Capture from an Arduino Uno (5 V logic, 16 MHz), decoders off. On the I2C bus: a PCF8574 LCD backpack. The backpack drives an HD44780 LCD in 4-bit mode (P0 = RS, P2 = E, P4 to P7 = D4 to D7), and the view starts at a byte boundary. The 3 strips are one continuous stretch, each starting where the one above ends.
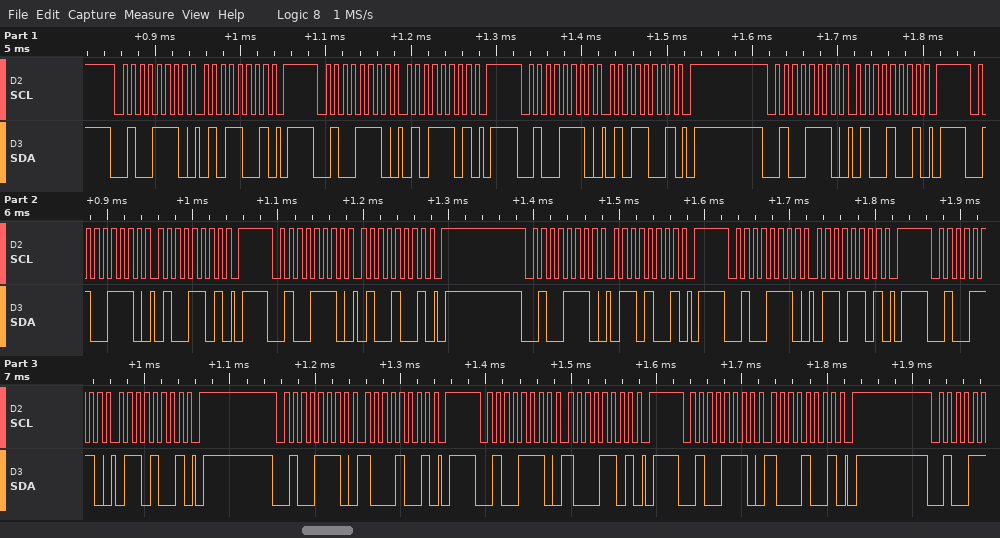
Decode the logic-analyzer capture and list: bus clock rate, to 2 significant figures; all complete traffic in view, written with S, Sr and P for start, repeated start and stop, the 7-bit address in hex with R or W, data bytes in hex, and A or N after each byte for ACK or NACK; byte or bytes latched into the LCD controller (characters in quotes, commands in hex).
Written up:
100 kHz
S 27W A 59 A P S 27W A 5D A P S 27W A 59 A P S 27W A 49 A P S 27W A 4D A P S 27W A 49 A P S 27W A 69 A P S 27W A 6D A P S 27W A 69 A P S 27W A 89 A P S 27W A 8D A P S 27W A 89 A P
'T' 'h'
